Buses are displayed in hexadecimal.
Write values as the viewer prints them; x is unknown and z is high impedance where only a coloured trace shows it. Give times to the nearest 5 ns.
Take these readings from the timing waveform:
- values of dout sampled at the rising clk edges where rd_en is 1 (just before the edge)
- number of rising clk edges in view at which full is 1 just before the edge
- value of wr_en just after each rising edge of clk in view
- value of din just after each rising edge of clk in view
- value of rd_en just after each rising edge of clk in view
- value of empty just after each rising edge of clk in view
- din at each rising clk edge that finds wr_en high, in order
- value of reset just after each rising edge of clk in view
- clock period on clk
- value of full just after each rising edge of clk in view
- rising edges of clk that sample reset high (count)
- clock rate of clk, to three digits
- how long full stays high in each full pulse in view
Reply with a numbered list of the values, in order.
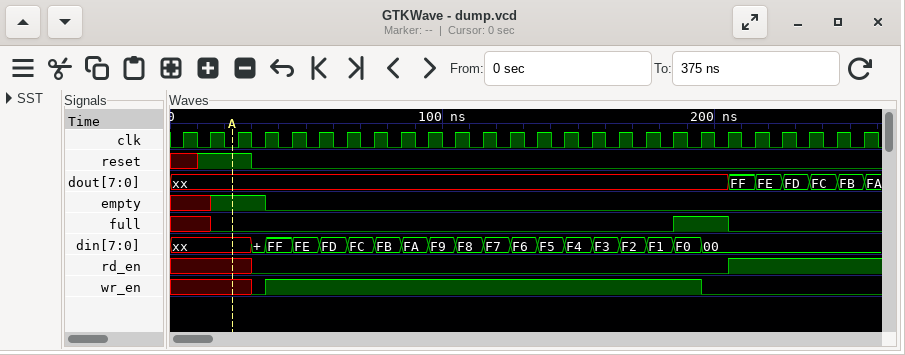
1. FF, FE, FD, FC, FB
2. 2
3. x x x 1 1 1 1 1 1 1 1 1 1 1 1 1 1 1 1 0 0 0 0 0 0 0
4. xx, xx, xx, FF, FE, FD, FC, FB, FA, F9, F8, F7, F6, F5, F4, F3, F2, F1, F0, 00, 00, 00, 00, 00, 00, 00
5. x x x 0 0 0 0 0 0 0 0 0 0 0 0 0 0 0 0 0 1 1 1 1 1 1
6. x 1 1 0 0 0 0 0 0 0 0 0 0 0 0 0 0 0 0 0 0 0 0 0 0 0
7. FF, FE, FD, FC, FB, FA, F9, F8, F7, F6, F5, F4, F3, F2, F1, F0
8. x 1 1 0 0 0 0 0 0 0 0 0 0 0 0 0 0 0 0 0 0 0 0 0 0 0
9. 10 ns
10. x 0 0 0 0 0 0 0 0 0 0 0 0 0 0 0 0 0 1 1 0 0 0 0 0 0
11. 2
12. 100 MHz
13. 20 ns
